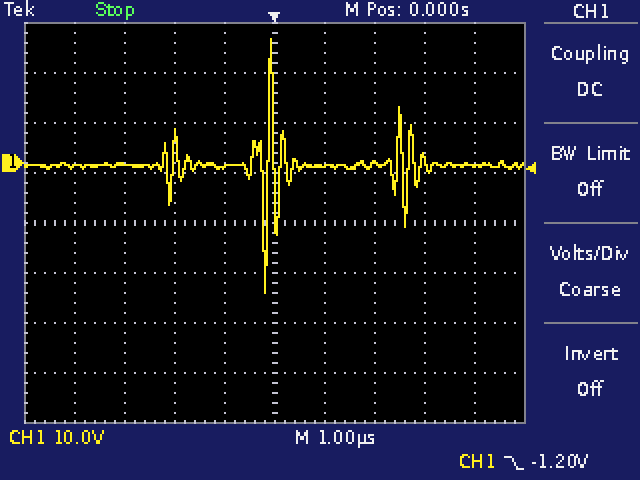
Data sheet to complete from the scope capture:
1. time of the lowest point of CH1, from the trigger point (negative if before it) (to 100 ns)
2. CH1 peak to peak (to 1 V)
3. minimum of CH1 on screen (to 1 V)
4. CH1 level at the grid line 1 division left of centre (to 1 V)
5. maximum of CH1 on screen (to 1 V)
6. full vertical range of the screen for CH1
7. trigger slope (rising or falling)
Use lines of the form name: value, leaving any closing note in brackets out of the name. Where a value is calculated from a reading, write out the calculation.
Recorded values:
time of the lowest point of CH1, from the trigger point (negative if before it): -200 ns
CH1 peak to peak: 25 V − (-26 V) = 51 V
minimum of CH1 on screen: -26 V
CH1 level at the grid line 1 division left of centre: -1 V
maximum of CH1 on screen: 25 V
full vertical range of the screen for CH1: 80 V
trigger slope: falling
